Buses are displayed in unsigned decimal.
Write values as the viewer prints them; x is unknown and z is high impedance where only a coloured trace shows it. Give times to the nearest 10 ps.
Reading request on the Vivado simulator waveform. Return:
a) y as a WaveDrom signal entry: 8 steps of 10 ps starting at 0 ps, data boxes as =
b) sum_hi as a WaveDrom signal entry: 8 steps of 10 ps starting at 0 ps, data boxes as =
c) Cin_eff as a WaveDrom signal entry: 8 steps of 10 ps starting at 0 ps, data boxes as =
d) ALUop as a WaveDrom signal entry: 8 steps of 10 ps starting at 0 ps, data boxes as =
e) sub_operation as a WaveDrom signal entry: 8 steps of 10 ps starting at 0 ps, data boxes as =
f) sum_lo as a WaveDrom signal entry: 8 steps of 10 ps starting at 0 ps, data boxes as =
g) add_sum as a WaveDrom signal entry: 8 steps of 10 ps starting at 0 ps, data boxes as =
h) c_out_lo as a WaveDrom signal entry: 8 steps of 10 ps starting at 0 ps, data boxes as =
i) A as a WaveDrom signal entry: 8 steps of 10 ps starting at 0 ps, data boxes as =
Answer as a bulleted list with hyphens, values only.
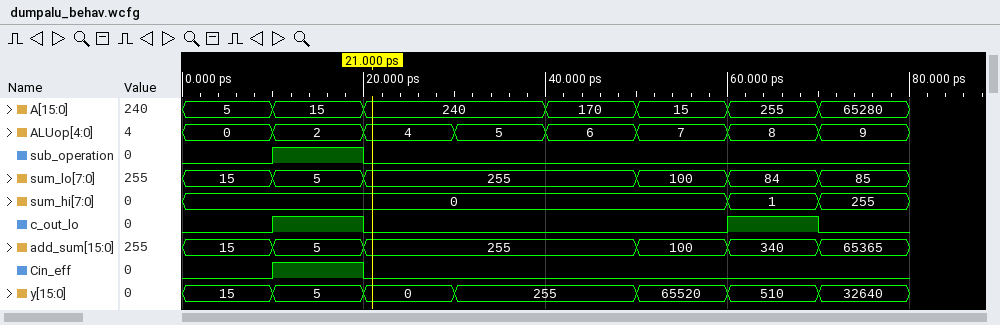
- {name: 'y', wave: '====.===', data: '15 5 0 255 65520 510 32640'}
- {name: 'sum_hi', wave: '=.....==', data: '0 1 255'}
- {name: 'Cin_eff', wave: '010.....'}
- {name: 'ALUop', wave: '========', data: '0 2 4 5 6 7 8 9'}
- {name: 'sub_operation', wave: '010.....'}
- {name: 'sum_lo', wave: '===..===', data: '15 5 255 100 84 85'}
- {name: 'add_sum', wave: '===..===', data: '15 5 255 100 340 65365'}
- {name: 'c_out_lo', wave: '010...10'}
- {name: 'A', wave: '===.====', data: '5 15 240 170 15 255 65280'}
